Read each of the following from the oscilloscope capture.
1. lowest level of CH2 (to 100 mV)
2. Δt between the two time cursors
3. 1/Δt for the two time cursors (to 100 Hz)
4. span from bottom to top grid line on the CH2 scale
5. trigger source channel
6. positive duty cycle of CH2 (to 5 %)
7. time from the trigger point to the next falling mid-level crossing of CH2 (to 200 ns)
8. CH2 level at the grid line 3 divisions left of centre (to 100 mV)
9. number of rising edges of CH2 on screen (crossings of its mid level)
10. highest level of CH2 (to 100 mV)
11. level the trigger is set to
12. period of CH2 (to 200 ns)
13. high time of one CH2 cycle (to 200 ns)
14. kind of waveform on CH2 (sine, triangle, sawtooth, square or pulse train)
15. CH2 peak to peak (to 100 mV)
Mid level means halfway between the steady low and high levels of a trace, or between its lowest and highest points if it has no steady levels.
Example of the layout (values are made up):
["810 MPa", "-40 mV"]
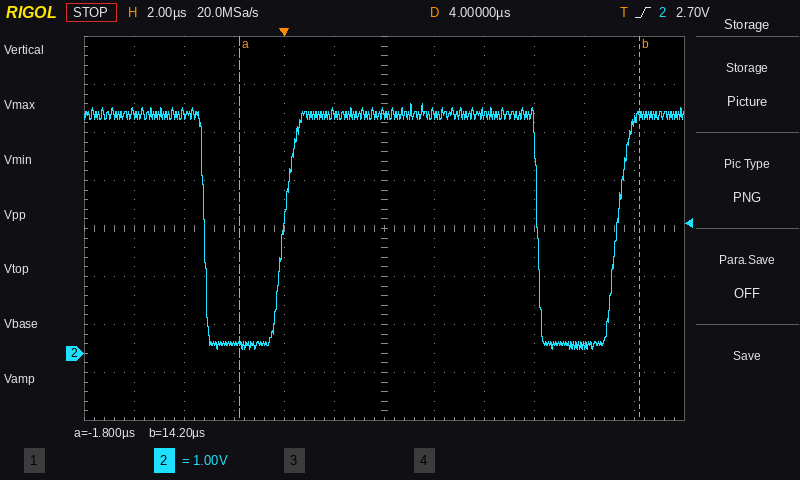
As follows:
["100 mV", "16.0 µs", "62.5 kHz", "8 V", "CH2", "75 %", "10.2 µs", "200 mV", "2", "5.2 V", "2.70 V", "13.4 µs", "10.2 µs", "pulse train", "5.1 V"]
